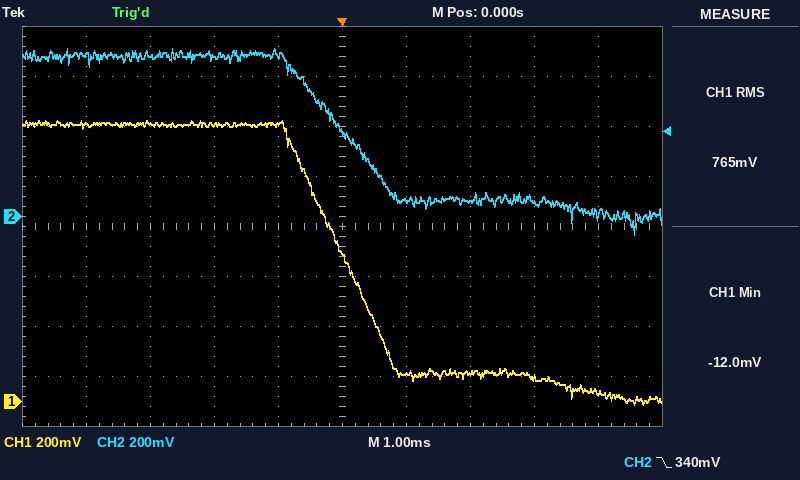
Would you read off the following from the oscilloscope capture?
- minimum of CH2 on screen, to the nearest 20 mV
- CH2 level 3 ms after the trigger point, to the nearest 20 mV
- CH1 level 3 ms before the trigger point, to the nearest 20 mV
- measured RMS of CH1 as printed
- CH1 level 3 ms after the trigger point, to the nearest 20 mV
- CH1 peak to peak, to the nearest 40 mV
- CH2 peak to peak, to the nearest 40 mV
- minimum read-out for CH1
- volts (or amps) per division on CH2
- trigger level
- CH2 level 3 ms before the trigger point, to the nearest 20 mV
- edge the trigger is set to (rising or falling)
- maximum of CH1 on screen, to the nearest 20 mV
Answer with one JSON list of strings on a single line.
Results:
["-80 mV", "60 mV", "1.12 V", "765 mV", "100 mV", "1.12 V", "760 mV", "-12.0 mV", "200 mV", "340 mV", "640 mV", "falling", "1.12 V"]
